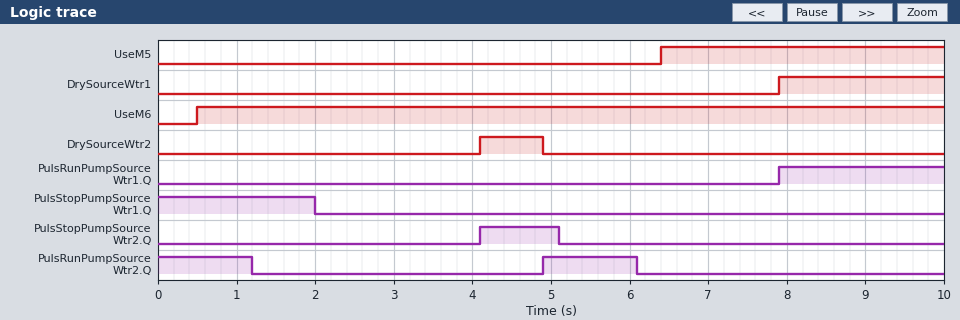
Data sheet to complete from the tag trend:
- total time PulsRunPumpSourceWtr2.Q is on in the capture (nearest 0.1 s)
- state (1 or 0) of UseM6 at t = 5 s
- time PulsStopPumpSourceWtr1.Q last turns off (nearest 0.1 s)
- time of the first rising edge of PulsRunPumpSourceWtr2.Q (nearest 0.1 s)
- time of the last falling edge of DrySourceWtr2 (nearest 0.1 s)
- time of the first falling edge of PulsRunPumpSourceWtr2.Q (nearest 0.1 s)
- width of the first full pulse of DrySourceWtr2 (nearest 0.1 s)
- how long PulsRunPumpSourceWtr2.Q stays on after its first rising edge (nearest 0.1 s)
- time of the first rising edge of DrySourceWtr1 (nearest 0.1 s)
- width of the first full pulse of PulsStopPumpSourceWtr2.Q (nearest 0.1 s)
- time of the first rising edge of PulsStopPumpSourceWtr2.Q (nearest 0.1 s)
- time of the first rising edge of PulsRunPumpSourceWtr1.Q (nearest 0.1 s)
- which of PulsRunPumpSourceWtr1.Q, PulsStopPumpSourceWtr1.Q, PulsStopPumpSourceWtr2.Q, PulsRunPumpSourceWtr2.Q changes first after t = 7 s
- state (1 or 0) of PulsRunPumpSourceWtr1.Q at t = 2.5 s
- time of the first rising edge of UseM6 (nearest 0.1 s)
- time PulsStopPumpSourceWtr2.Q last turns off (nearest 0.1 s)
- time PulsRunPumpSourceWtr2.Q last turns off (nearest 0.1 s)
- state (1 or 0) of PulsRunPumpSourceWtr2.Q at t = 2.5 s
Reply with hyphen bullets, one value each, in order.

- 2.4 s
- 1
- 2.0 s
- 4.9 s
- 4.9 s
- 1.2 s
- 0.8 s
- 1.2 s
- 7.9 s
- 1.0 s
- 4.1 s
- 7.9 s
- PulsRunPumpSourceWtr1.Q
- 0
- 0.5 s
- 5.1 s
- 6.1 s
- 0
